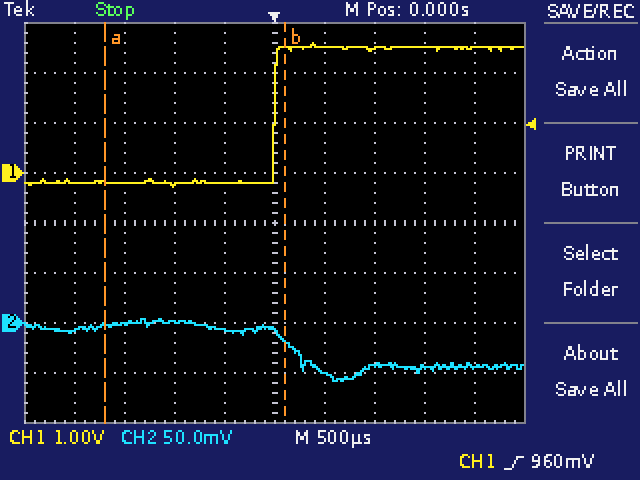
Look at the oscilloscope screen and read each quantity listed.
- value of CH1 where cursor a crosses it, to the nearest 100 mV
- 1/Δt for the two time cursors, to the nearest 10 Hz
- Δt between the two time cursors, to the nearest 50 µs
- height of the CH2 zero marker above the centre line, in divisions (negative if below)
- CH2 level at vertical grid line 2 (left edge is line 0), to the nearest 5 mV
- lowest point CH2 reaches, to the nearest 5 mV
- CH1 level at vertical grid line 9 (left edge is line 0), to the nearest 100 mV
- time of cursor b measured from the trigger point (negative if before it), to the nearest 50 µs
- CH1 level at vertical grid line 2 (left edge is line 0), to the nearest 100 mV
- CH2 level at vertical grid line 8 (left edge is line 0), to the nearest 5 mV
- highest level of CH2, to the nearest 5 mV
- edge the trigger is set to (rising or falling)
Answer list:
-200 mV
560 Hz
1.80 ms
-2.0 div
0 mV
-60 mV
2.5 V
+100 µs
-200 mV
-45 mV
5 mV
rising
